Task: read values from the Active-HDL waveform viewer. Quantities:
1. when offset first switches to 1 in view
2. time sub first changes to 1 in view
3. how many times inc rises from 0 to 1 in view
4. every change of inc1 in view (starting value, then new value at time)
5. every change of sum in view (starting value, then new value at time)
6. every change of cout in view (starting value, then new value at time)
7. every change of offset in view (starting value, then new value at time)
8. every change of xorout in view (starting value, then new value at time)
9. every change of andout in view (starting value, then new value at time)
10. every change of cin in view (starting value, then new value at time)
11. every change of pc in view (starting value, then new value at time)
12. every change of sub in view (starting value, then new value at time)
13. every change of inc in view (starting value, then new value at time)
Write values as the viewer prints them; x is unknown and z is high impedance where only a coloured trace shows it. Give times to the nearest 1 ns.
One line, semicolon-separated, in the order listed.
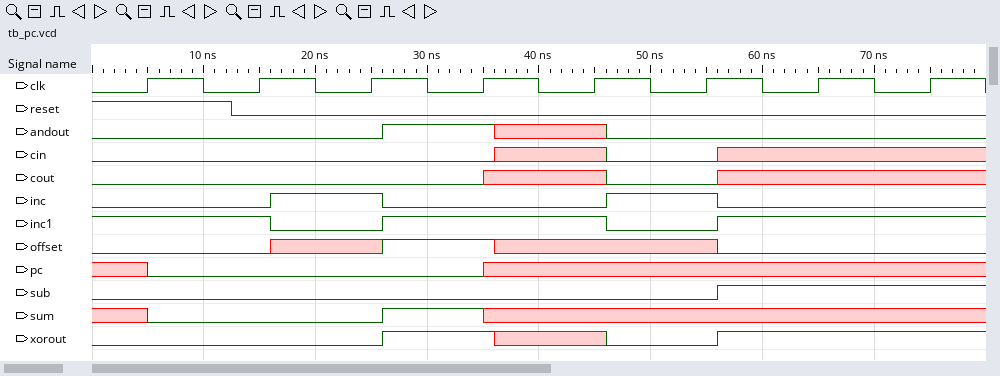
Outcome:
26 ns; 56 ns; 2; 1, 0 at 16 ns, 1 at 26 ns, 0 at 46 ns, 1 at 56 ns; x, 0 at 5 ns, 1 at 26 ns, x at 35 ns; 0, x at 35 ns, 0 at 46 ns, x at 56 ns; 0, x at 16 ns, 1 at 26 ns, x at 36 ns, 0 at 56 ns; 0, 1 at 26 ns, x at 36 ns, 0 at 46 ns, 1 at 56 ns; 0, 1 at 26 ns, x at 36 ns, 0 at 46 ns; 0, x at 36 ns, 0 at 46 ns, x at 56 ns; x, 0 at 5 ns, x at 35 ns; 0, 1 at 56 ns; 0, 1 at 16 ns, 0 at 26 ns, 1 at 46 ns, 0 at 56 ns
